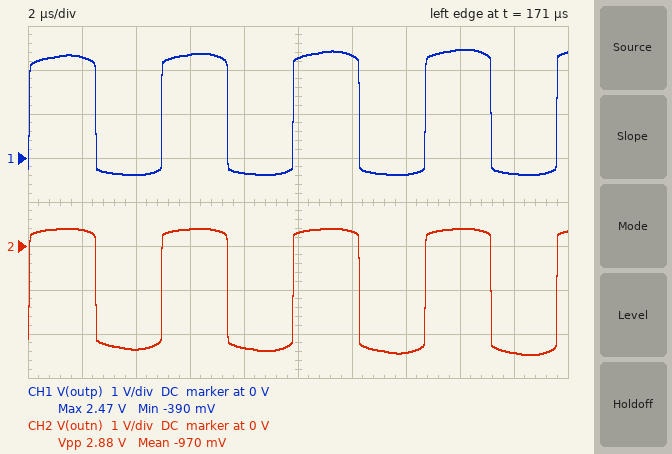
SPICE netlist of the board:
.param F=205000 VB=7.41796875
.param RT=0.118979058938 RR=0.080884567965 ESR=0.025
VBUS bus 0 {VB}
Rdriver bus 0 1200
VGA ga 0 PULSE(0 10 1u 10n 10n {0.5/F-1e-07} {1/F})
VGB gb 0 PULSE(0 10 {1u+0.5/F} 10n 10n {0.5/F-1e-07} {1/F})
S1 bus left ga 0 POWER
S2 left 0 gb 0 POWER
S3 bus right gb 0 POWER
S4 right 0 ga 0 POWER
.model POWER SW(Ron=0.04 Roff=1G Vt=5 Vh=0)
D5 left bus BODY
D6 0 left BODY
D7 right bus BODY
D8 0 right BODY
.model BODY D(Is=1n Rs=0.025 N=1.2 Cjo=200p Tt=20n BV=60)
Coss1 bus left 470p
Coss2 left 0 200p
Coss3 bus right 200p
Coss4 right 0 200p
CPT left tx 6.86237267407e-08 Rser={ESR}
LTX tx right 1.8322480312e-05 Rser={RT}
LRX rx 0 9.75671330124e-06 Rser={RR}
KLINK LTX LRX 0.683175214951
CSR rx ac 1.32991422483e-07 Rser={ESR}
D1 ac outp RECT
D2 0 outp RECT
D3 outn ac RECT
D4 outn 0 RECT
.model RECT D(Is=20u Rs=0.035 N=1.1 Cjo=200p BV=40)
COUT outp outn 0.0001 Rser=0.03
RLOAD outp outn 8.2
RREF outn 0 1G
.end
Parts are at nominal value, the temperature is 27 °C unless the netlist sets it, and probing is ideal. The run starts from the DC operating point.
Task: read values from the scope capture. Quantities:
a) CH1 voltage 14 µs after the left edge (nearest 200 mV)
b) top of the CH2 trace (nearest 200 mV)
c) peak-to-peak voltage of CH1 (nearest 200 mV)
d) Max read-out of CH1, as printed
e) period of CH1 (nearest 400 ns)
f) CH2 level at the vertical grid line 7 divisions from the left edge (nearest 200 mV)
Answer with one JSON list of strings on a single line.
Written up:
["-400 mV", "400 mV", "2.8 V", "2.47 V", "4.8 µs", "-2.4 V"]
